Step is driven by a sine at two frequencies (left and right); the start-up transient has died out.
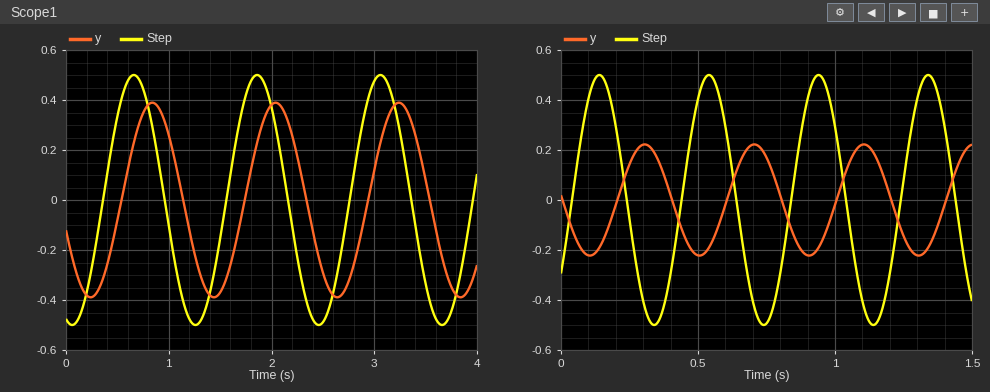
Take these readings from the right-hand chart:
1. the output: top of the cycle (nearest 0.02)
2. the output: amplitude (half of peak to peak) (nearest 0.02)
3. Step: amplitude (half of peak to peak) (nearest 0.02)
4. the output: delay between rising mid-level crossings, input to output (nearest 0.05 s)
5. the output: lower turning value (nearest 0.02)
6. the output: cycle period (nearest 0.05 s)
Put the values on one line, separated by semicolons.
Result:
0.22; 0.22; 0.50; 0.15 s; -0.22; 0.40 s
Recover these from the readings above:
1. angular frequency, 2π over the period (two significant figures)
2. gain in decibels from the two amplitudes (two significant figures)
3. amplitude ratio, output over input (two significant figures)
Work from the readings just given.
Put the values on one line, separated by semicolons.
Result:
16 rad/s; -7.1 dB; 0.44
